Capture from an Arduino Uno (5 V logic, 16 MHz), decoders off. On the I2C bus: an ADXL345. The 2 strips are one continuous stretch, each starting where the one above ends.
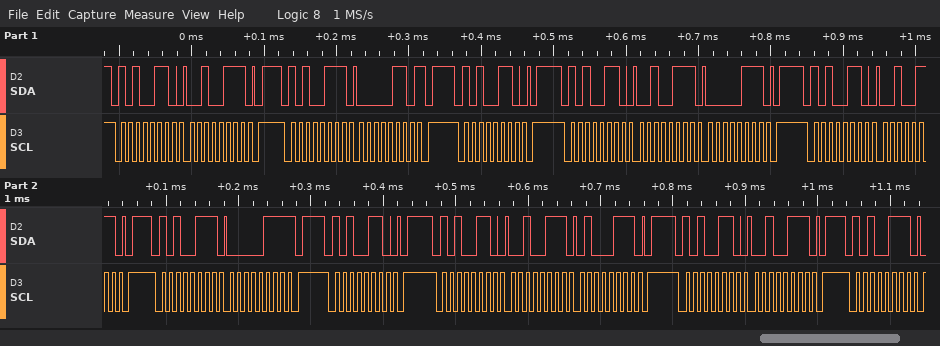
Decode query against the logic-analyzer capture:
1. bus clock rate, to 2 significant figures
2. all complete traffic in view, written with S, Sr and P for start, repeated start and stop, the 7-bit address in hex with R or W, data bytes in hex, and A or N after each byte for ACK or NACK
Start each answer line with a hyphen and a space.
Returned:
- 100 kHz
- S 53W A 27 A P S 53R A 06 N P S 53W A P S 53W A 27 A 07 A P S 53W A 27 A P S 53R A 07 N P S 53W A P S 53W A 27 A 47 A P S 53W A 27 A P S 53R A
